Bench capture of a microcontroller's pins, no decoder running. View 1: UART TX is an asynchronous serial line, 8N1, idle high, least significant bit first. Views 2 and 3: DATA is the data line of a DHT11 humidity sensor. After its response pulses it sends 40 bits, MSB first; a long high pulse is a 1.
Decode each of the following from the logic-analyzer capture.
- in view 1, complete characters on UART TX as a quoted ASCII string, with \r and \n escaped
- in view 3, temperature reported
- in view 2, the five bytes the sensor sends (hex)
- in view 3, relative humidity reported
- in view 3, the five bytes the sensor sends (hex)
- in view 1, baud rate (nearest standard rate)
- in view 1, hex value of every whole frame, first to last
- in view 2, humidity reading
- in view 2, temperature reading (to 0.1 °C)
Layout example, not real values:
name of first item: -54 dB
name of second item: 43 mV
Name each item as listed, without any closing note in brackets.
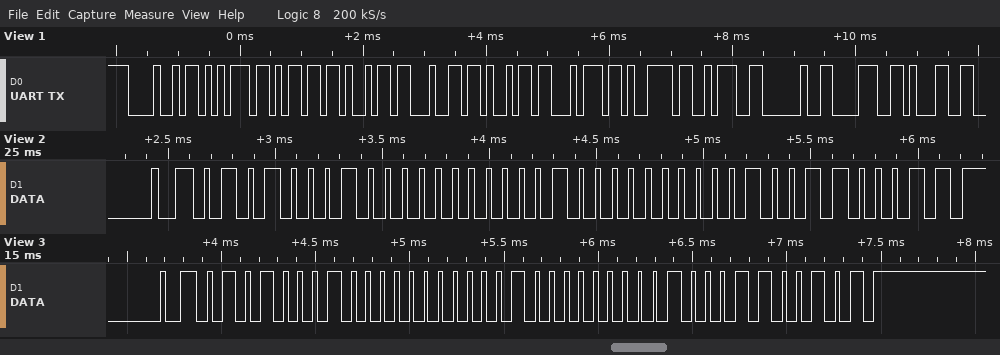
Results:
in view 1, complete characters on UART TX as a quoted ASCII string, with \r and \n escaped: "Humidity: 81"
in view 3, temperature reported: 16.4 °C
in view 2, the five bytes the sensor sends: 51 00 10 02 63
in view 3, relative humidity reported: 81 %
in view 3, the five bytes the sensor sends: 51 00 10 04 65
in view 1, baud rate: 9600 baud
in view 1, hex value of every whole frame, first to last: 48 75 6D 69 64 69 74 79 3A 20 38 31
in view 2, humidity reading: 81 %
in view 2, temperature reading: 16.2 °C
